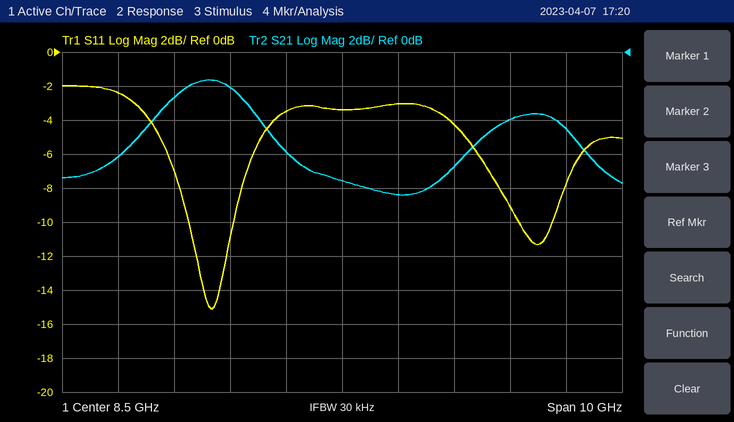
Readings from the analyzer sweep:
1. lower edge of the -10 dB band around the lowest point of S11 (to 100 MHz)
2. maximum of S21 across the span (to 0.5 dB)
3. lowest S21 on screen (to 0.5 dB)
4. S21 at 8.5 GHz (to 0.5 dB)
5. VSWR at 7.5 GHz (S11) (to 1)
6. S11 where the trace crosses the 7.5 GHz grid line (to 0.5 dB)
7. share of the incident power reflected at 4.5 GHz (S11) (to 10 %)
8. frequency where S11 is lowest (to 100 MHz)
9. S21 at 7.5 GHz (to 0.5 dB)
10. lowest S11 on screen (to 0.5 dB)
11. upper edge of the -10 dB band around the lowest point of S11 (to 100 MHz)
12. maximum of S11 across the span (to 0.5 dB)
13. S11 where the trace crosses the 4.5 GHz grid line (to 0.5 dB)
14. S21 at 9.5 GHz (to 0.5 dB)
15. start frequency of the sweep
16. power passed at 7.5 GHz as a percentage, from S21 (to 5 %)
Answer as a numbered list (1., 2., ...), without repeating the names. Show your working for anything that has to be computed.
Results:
1. 5.8 GHz
2. -1.5 dB
3. -8.5 dB
4. -7.5 dB
5. |Γ| = 10^(-3.5/20) = 0.6683; VSWR = (1 + 0.6683)/(1 − 0.6683) ≈ 5
6. -3.5 dB
7. 10^(-2.5/10) ≈ 56.2 %, so 60 % to the nearest 10 %
8. 6.2 GHz
9. -6.0 dB
10. -15.0 dB
11. 6.6 GHz
12. -2.0 dB
13. -2.5 dB
14. -8.5 dB
15. 3.5 GHz
16. 10^(-6/10) ≈ 25 %
